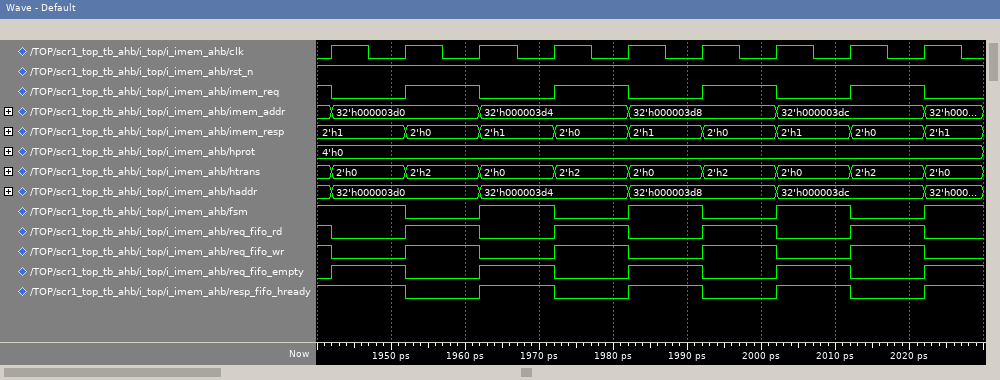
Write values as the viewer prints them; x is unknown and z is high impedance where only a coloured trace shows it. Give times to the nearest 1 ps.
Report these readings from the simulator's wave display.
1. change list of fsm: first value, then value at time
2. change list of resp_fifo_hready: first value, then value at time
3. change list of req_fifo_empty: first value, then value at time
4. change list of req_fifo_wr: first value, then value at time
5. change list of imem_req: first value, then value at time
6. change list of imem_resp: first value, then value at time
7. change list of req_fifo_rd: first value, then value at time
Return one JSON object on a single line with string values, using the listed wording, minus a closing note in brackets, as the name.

{"change list of fsm: first value, then value at time": "1, 0 at 1952 ps, 1 at 1962 ps, 0 at 1972 ps, 1 at 1982 ps, 0 at 1992 ps, 1 at 2002 ps, 0 at 2012 ps, 1 at 2022 ps", "change list of resp_fifo_hready: first value, then value at time": "1, 0 at 1952 ps, 1 at 1962 ps, 0 at 1972 ps, 1 at 1982 ps, 0 at 1992 ps, 1 at 2002 ps, 0 at 2012 ps, 1 at 2022 ps", "change list of req_fifo_empty: first value, then value at time": "0, 1 at 1942 ps, 0 at 1952 ps, 1 at 1962 ps, 0 at 1972 ps, 1 at 1982 ps, 0 at 1992 ps, 1 at 2002 ps, 0 at 2012 ps, 1 at 2022 ps", "change list of req_fifo_wr: first value, then value at time": "1, 0 at 1942 ps, 1 at 1952 ps, 0 at 1962 ps, 1 at 1972 ps, 0 at 1982 ps, 1 at 1992 ps, 0 at 2002 ps, 1 at 2012 ps, 0 at 2022 ps", "change list of imem_req: first value, then value at time": "1, 0 at 1942 ps, 1 at 1952 ps, 0 at 1962 ps, 1 at 1972 ps, 0 at 1982 ps, 1 at 1992 ps, 0 at 2002 ps, 1 at 2012 ps, 0 at 2022 ps", "change list of imem_resp: first value, then value at time": "2'h1, 2'h0 at 1952 ps, 2'h1 at 1962 ps, 2'h0 at 1972 ps, 2'h1 at 1982 ps, 2'h0 at 1992 ps, 2'h1 at 2002 ps, 2'h0 at 2012 ps, 2'h1 at 2022 ps", "change list of req_fifo_rd: first value, then value at time": "1, 0 at 1942 ps, 1 at 1952 ps, 0 at 1962 ps, 1 at 1972 ps, 0 at 1982 ps, 1 at 1992 ps, 0 at 2002 ps, 1 at 2012 ps, 0 at 2022 ps"}
